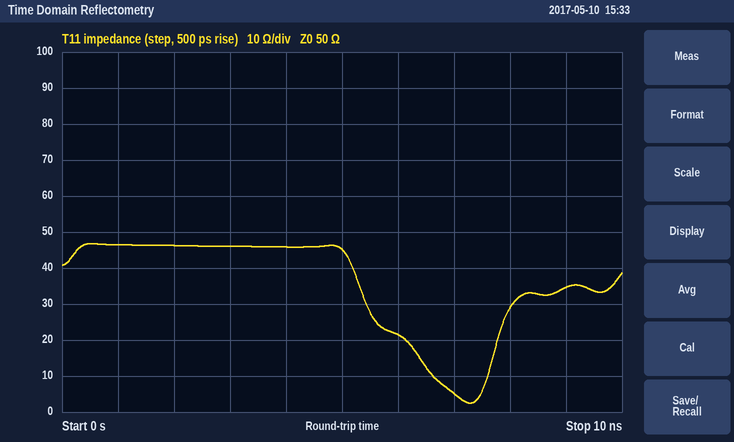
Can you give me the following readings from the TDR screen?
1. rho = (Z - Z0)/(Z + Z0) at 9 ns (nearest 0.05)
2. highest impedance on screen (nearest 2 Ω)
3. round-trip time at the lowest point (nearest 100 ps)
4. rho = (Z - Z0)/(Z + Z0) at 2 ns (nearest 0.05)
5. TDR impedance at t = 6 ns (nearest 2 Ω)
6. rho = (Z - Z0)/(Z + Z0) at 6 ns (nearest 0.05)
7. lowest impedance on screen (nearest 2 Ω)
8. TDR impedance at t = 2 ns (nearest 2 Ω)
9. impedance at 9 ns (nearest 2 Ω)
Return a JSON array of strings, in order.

["-0.20", "46 Ω", "7.3 ns", "-0.05", "22 Ω", "-0.40", "2 Ω", "46 Ω", "34 Ω"]
